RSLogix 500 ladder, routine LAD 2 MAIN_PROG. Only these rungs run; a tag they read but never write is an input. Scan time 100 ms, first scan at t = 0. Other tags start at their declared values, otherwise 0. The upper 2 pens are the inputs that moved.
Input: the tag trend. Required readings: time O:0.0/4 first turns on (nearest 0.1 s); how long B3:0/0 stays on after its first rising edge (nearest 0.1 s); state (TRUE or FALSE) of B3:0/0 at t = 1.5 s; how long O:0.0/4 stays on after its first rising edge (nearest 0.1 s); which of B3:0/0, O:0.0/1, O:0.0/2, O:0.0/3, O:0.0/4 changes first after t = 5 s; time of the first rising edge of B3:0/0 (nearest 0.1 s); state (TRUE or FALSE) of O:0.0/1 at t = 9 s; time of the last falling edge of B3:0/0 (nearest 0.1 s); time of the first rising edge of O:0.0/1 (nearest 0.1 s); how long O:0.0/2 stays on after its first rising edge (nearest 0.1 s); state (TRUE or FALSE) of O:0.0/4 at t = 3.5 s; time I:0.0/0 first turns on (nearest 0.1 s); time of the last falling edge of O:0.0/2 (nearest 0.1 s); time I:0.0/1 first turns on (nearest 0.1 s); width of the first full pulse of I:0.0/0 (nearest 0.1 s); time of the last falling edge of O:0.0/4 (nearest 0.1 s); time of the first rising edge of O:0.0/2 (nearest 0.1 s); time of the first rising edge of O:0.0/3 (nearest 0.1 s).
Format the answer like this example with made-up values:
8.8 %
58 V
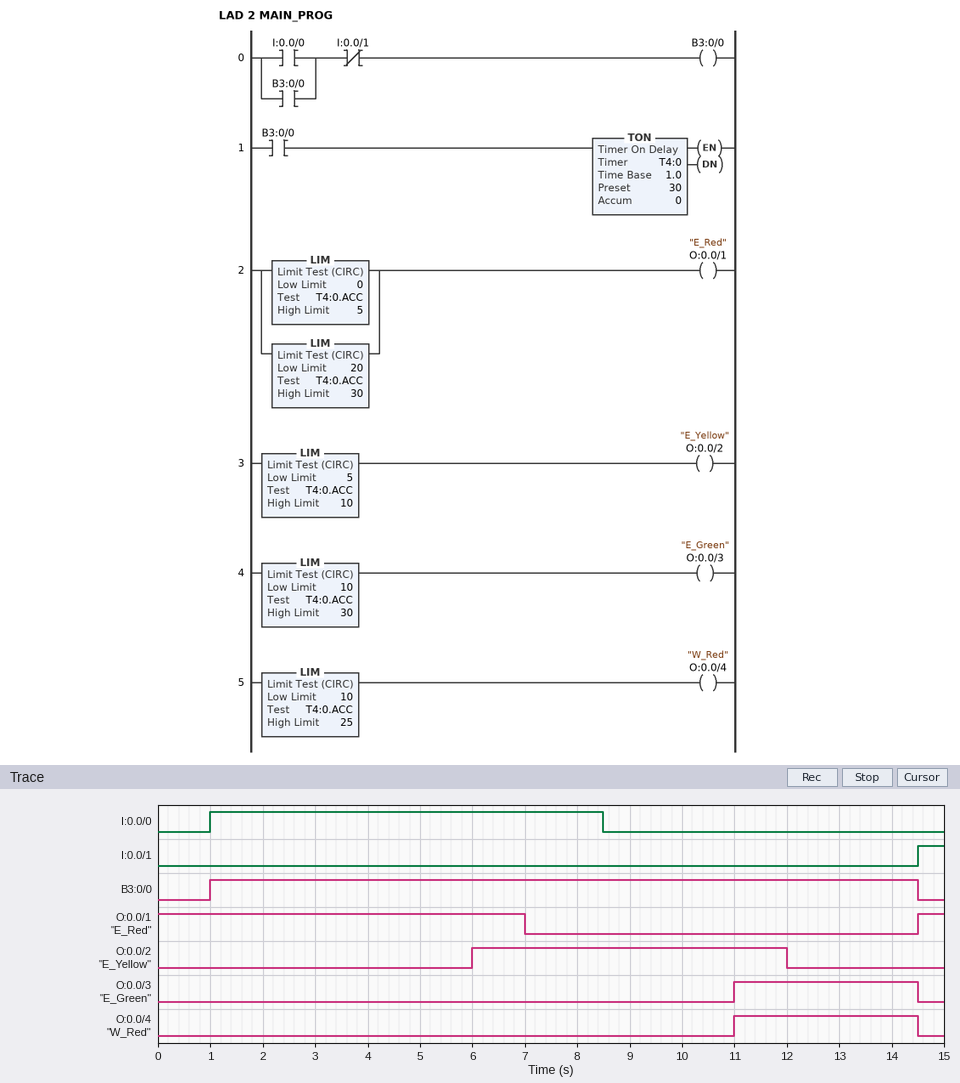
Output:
11.0 s
13.5 s
TRUE
3.5 s
O:0.0/2
1.0 s
FALSE
14.5 s
14.5 s
6.0 s
FALSE
1.0 s
12.0 s
14.5 s
7.5 s
14.5 s
6.0 s
11.0 s
